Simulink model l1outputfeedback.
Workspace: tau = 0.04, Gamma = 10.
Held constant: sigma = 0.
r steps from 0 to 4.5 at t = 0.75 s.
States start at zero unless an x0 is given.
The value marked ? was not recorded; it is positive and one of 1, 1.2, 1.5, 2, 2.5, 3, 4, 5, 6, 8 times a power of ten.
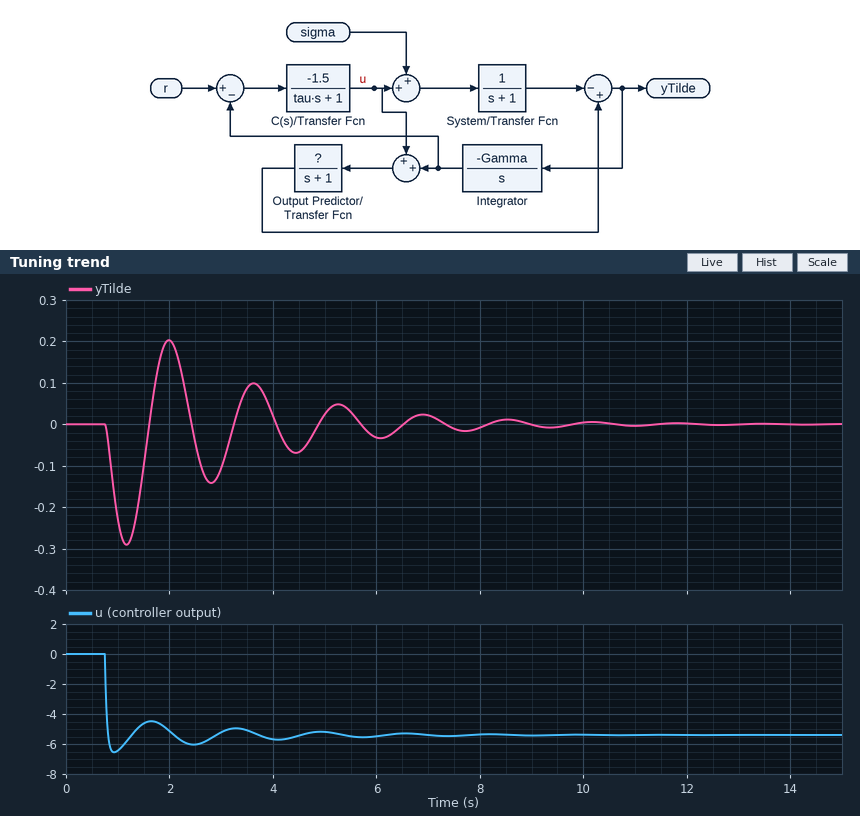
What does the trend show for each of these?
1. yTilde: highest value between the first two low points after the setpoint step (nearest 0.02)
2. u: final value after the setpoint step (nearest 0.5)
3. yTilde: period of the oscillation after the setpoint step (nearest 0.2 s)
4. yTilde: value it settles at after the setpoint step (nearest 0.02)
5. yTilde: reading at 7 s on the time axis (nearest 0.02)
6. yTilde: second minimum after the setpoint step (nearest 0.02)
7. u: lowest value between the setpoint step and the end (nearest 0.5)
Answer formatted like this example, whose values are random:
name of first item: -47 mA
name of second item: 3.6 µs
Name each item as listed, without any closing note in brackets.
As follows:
yTilde: highest value between the first two low points after the setpoint step: 0.20
u: final value after the setpoint step: -5.5
yTilde: period of the oscillation after the setpoint step: 1.6 s
yTilde: value it settles at after the setpoint step: 0.00
yTilde: reading at 7 s on the time axis: 0.02
yTilde: second minimum after the setpoint step: -0.14
u: lowest value between the setpoint step and the end: -6.5
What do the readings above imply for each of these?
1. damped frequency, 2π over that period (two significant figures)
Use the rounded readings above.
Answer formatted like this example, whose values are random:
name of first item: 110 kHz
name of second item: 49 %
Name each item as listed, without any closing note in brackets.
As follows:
damped frequency, 2π over that period: 3.9 rad/s
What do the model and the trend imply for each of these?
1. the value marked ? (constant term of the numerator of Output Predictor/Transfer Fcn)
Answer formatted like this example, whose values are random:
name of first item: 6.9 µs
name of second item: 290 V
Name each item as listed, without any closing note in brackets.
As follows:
the value marked ?: 1.2
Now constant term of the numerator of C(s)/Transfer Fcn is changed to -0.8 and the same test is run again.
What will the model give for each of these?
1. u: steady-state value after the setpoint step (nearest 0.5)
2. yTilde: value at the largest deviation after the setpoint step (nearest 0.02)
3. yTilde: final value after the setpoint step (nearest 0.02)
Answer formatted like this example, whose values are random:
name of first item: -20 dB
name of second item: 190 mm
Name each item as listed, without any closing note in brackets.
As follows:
u: steady-state value after the setpoint step: -3.0
yTilde: value at the largest deviation after the setpoint step: -0.16
yTilde: final value after the setpoint step: 0.00
